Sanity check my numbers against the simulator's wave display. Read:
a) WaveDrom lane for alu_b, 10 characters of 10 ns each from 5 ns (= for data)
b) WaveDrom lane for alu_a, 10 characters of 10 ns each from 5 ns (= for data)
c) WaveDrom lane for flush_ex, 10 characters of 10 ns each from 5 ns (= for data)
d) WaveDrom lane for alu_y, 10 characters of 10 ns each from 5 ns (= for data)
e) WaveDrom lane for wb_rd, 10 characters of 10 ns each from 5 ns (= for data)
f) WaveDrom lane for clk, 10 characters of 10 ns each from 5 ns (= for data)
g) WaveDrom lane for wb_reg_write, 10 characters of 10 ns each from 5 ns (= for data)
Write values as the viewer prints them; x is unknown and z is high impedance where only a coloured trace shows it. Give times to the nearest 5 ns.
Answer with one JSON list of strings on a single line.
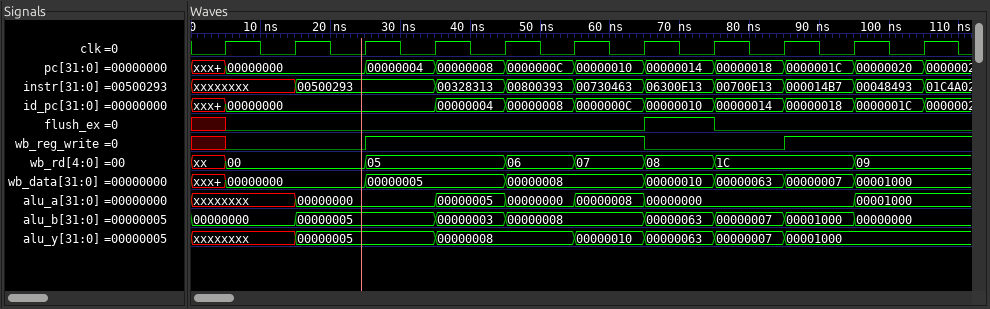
["{name: 'alu_b', wave: '==.==.====', data: '00000000 00000005 00000003 00000008 00000063 00000007 00001000 00000000'}", "{name: 'alu_a', wave: 'x=.====..=', data: '00000000 00000005 00000000 00000008 00000000 00001000'}", "{name: 'flush_ex', wave: '0.....10..'}", "{name: 'alu_y', wave: 'x=.=.====.', data: '00000005 00000008 00000010 00000063 00000007 00001000'}", "{name: 'wb_rd', wave: '=.=.====.=', data: '00 05 06 07 08 1C 09'}", "{name: 'clk', wave: 'p.........'}", "{name: 'wb_reg_write', wave: '0.1...0.1.'}"]
